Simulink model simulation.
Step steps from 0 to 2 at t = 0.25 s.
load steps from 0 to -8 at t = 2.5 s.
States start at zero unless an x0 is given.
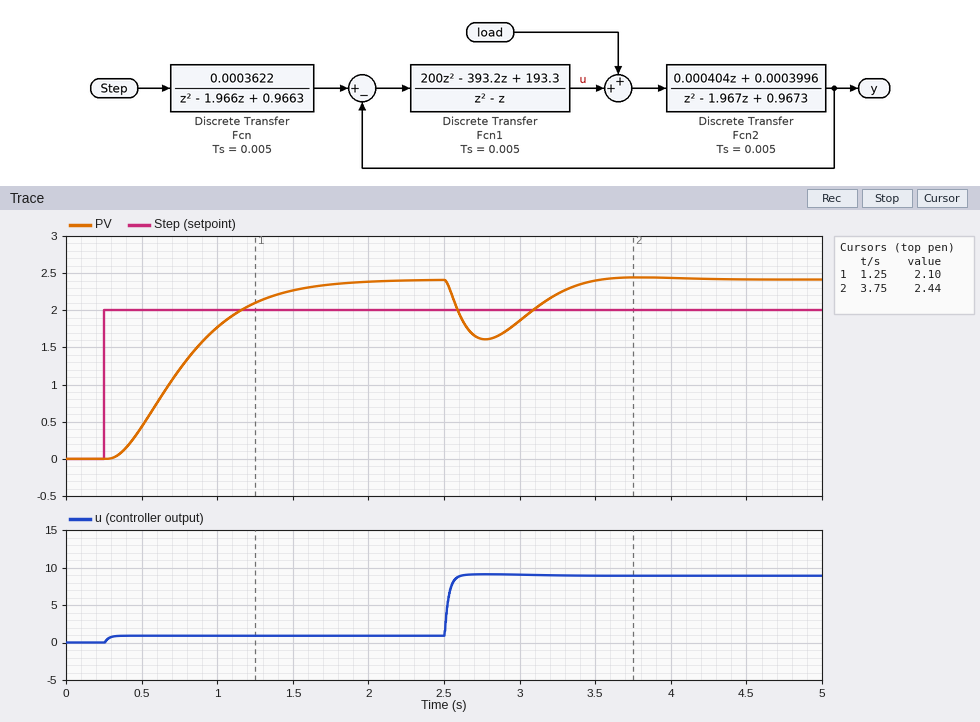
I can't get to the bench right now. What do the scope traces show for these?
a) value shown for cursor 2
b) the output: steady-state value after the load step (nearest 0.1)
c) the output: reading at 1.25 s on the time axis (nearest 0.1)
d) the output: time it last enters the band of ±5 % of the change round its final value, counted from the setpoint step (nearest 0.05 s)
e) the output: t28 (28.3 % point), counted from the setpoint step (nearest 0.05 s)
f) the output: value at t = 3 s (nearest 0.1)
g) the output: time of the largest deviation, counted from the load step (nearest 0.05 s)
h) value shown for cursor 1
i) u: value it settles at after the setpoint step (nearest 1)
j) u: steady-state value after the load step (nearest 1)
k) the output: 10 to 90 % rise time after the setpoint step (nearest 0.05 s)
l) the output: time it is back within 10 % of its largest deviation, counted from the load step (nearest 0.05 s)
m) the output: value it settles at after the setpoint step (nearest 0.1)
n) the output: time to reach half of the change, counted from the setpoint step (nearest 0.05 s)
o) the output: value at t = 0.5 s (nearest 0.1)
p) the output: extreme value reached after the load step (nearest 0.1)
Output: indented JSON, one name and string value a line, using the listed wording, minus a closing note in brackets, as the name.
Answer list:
{
  "value shown for cursor 2": "2.44",
  "the output: steady-state value after the load step": "2.4",
  "the output: reading at 1.25 s on the time axis": "2.1",
  "the output: time it last enters the band of ±5 % of the change round its final value, counted from the setpoint step": "1.30 s",
  "the output: t28 (28.3 % point), counted from the setpoint step": "0.35 s",
  "the output: value at t = 3 s": "1.9",
  "the output: time of the largest deviation, counted from the load step": "0.25 s",
  "value shown for cursor 1": "2.10",
  "u: value it settles at after the setpoint step": "1",
  "u: steady-state value after the load step": "9",
  "the output: 10 to 90 % rise time after the setpoint step": "0.90 s",
  "the output: time it is back within 10 % of its largest deviation, counted from the load step": "0.90 s",
  "the output: value it settles at after the setpoint step": "2.4",
  "the output: time to reach half of the change, counted from the setpoint step": "0.50 s",
  "the output: value at t = 0.5 s": "0.4",
  "the output: extreme value reached after the load step": "1.6"
}
